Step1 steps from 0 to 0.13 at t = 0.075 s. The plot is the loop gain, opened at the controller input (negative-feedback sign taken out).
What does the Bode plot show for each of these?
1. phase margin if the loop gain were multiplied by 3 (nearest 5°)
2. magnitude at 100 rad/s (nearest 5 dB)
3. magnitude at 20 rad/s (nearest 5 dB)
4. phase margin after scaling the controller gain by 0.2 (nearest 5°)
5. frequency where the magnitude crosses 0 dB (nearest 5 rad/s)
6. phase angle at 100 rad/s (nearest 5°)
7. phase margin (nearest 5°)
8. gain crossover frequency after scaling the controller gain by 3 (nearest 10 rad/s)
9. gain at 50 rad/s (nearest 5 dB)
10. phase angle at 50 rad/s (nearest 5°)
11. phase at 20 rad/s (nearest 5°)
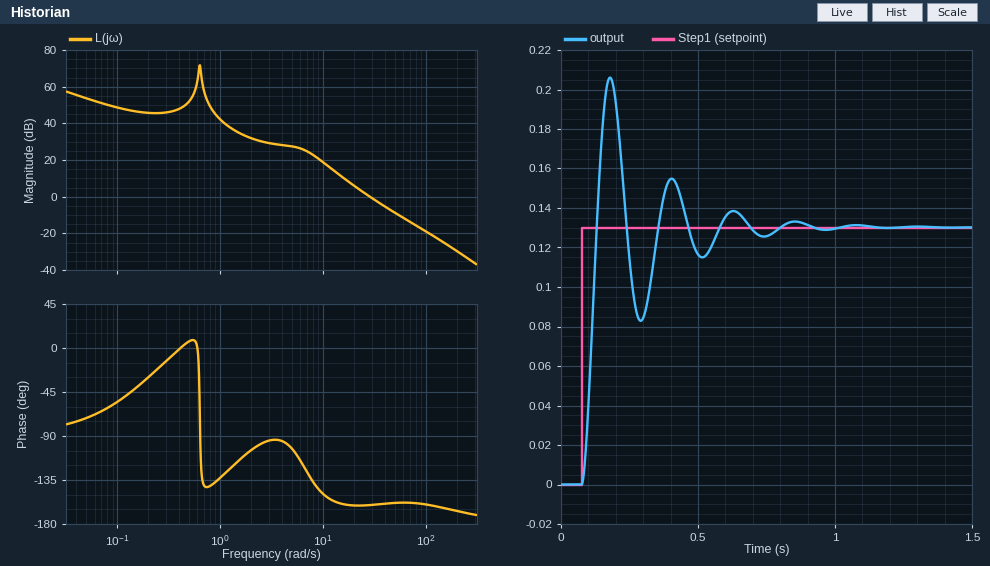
20°
-20 dB
5 dB
25°
30 rad/s
-160°
20°
50 rad/s
-10 dB
-160°
-160°
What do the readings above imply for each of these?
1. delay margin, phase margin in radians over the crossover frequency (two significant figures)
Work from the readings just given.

0.012 s
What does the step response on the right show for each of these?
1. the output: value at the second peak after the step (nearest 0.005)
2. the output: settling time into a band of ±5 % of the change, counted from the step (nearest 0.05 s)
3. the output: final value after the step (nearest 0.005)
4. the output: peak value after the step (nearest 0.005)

0.155
0.60 s
0.130
0.205
